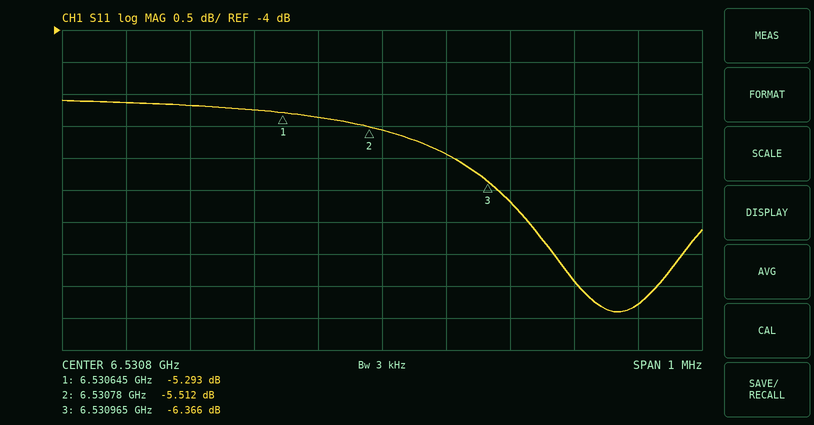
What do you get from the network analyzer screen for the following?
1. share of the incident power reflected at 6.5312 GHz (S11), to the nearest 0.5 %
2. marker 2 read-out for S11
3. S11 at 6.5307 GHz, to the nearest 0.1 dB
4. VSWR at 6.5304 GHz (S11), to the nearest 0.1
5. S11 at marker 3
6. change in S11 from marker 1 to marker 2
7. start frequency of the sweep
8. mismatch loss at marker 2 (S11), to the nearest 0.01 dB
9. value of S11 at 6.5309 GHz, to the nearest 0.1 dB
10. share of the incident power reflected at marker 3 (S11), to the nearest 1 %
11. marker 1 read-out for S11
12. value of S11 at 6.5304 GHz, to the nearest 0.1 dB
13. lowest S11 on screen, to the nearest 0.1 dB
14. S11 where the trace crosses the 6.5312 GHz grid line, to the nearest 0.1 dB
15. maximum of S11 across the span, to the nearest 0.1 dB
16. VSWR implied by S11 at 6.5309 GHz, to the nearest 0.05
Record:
15.0 %
-5.512 dB
-5.4 dB
3.5
-6.366 dB
-0.219 dB
6.5303 GHz
1.43 dB
-5.9 dB
23 %
-5.293 dB
-5.1 dB
-8.4 dB
-8.3 dB
-5.1 dB
3.05
